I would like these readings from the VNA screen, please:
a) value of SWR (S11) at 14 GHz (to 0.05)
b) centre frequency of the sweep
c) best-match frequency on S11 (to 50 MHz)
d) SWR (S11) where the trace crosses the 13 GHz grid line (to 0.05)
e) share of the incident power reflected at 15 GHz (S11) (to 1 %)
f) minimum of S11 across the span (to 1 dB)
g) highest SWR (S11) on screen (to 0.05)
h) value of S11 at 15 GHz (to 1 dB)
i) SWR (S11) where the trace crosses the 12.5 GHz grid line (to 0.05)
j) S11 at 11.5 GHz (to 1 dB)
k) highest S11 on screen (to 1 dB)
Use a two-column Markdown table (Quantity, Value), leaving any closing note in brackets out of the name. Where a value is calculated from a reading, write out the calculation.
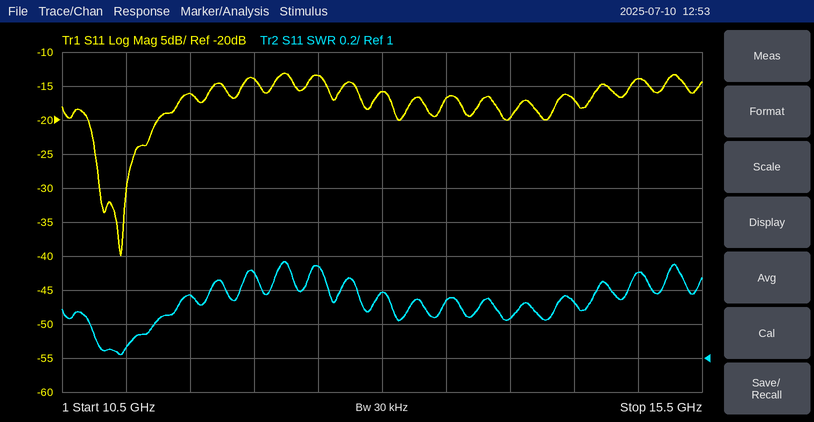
| Quantity | Value |
|---|---|
| value of SWR (S11) at 14 GHz | 1.25 |
| centre frequency of the sweep | 13 GHz |
| best-match frequency on S11 | 10.95 GHz |
| SWR (S11) where the trace crosses the 13 GHz grid line | 1.40 |
| share of the incident power reflected at 15 GHz (S11) | 10^(-14/10) ≈ 4 % |
| minimum of S11 across the span | -40 dB |
| highest SWR (S11) on screen | 1.55 |
| value of S11 at 15 GHz | -14 dB |
| SWR (S11) where the trace crosses the 12.5 GHz grid line | 1.55 |
| S11 at 11.5 GHz | -16 dB |
| highest S11 on screen | -13 dB |
